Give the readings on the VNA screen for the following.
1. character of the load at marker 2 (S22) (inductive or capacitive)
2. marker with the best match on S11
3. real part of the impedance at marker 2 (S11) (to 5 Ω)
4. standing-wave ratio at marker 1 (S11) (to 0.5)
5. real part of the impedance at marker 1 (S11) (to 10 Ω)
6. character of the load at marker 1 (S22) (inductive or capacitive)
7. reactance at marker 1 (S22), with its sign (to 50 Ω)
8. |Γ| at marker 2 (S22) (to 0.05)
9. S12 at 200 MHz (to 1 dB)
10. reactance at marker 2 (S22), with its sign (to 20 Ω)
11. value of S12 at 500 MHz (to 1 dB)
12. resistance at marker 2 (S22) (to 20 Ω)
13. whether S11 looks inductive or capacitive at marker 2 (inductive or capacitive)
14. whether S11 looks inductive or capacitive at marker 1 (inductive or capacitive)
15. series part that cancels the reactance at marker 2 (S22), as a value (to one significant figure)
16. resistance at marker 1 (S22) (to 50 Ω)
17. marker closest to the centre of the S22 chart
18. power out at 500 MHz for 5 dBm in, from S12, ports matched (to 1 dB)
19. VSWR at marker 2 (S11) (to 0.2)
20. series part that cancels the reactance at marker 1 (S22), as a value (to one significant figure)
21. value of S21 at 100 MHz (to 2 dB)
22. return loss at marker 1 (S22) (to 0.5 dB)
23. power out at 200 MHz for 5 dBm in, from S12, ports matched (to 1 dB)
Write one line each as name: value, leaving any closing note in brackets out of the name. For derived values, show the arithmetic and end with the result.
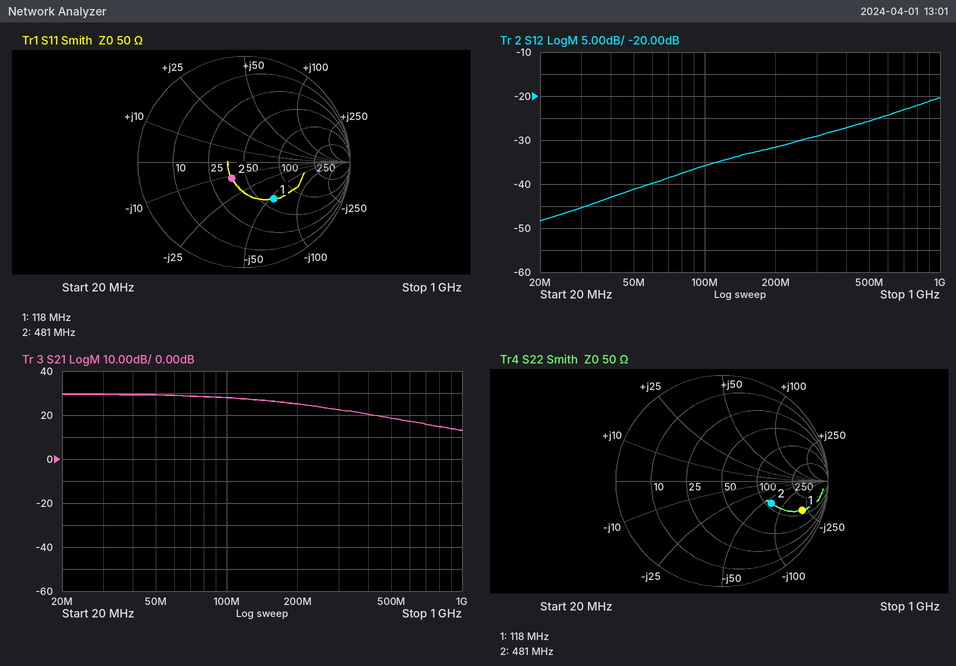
character of the load at marker 2 (S22): capacitive
marker with the best match on S11: marker 2
real part of the impedance at marker 2 (S11): 40 Ω
standing-wave ratio at marker 1 (S11): 2.5
real part of the impedance at marker 1 (S11): 60 Ω
character of the load at marker 1 (S22): capacitive
reactance at marker 1 (S22), with its sign: -200 Ω
|Γ| at marker 2 (S22): 0.50
S12 at 200 MHz: -32 dB
reactance at marker 2 (S22), with its sign: -60 Ω
value of S12 at 500 MHz: -26 dB
resistance at marker 2 (S22): 120 Ω
whether S11 looks inductive or capacitive at marker 2: capacitive
whether S11 looks inductive or capacitive at marker 1: capacitive
series part that cancels the reactance at marker 2 (S22), as a value: L = 60 Ω/(2π × 481 MHz) ≈ 20 nH
resistance at marker 1 (S22): 150 Ω
marker closest to the centre of the S22 chart: marker 2
power out at 500 MHz for 5 dBm in, from S12, ports matched: 5 dBm + (-26 dB) = -21 dBm
VSWR at marker 2 (S11): 1.4
series part that cancels the reactance at marker 1 (S22), as a value: L = 200 Ω/(2π × 118 MHz) ≈ 270 nH, so 300 nH to one significant figure
value of S21 at 100 MHz: 28 dB
return loss at marker 1 (S22): 2.0 dB
power out at 200 MHz for 5 dBm in, from S12, ports matched: 5 dBm + (-32 dB) = -27 dBm
